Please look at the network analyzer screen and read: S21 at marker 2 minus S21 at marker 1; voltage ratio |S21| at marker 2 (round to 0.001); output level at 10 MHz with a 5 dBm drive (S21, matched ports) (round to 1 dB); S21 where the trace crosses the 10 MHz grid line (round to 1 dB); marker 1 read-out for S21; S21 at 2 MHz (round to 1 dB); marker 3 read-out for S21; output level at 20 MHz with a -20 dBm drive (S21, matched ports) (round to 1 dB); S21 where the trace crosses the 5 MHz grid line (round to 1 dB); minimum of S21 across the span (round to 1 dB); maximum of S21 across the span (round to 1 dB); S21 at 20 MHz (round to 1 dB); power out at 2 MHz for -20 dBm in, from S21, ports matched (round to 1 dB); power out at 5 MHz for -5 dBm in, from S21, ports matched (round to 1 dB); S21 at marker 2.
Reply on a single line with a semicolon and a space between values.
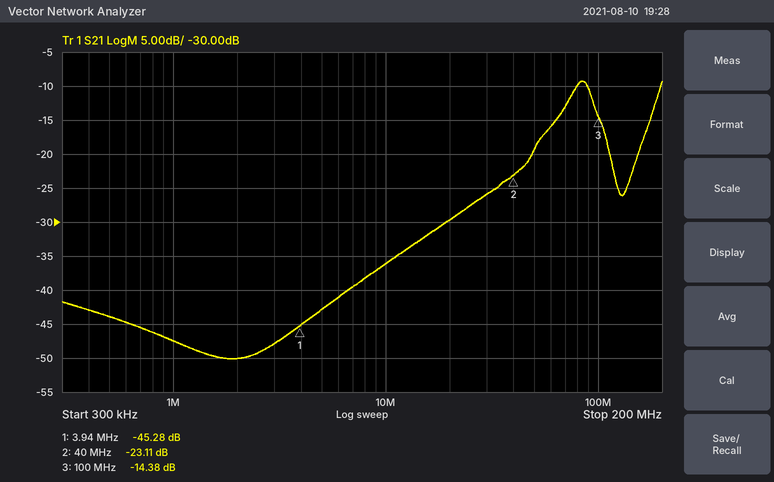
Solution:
22.17 dB; 0.070; -31 dBm; -36 dB; -45.28 dB; -50 dB; -14.38 dB; -50 dBm; -43 dB; -50 dB; -9 dB; -30 dB; -70 dBm; -48 dBm; -23.11 dB
